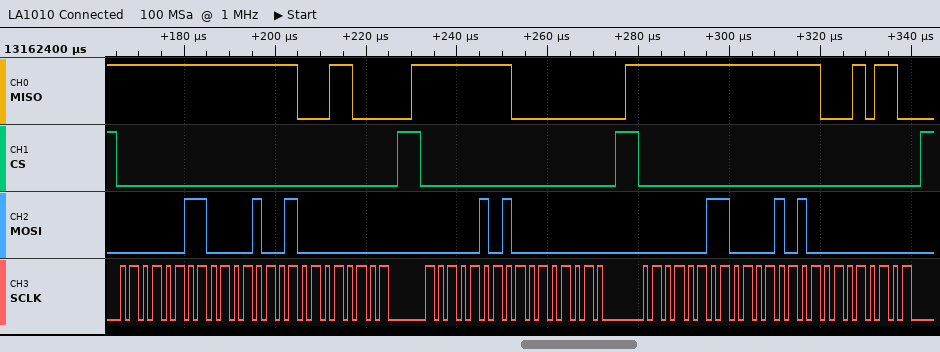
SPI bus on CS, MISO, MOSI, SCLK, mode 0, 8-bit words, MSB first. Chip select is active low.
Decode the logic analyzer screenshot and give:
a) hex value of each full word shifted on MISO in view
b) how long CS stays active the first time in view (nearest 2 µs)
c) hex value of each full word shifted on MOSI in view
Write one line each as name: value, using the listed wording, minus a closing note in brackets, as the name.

hex value of each full word shifted on MISO in view: FF, FF, 18, FF, 00, FF, FF, 16
how long CS stays active the first time in view: 62 µs
hex value of each full word shifted on MOSI in view: 03, 09, 00, 05, 00, 03, 0A, 00
